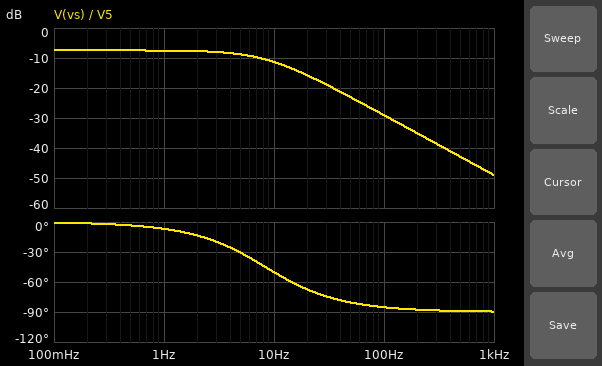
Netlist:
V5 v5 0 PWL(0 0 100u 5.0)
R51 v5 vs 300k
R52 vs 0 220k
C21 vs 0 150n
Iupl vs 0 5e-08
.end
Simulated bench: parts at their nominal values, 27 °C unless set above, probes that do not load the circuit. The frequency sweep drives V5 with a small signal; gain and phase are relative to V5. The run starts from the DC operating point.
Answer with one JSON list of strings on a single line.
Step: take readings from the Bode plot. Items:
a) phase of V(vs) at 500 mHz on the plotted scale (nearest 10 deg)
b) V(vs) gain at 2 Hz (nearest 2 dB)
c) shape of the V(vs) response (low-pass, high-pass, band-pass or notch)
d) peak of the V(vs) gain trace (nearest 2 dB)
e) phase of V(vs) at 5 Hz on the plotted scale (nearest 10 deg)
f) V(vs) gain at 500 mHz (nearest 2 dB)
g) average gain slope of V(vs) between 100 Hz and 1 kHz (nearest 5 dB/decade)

["0 deg", "-8 dB", "low-pass", "-8 dB", "-30 deg", "-8 dB", "-20 dB/decade"]
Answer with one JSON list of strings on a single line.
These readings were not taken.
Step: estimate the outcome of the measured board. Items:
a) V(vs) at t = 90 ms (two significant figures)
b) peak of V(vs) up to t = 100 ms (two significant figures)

["2.1 V", "2.1 V"]
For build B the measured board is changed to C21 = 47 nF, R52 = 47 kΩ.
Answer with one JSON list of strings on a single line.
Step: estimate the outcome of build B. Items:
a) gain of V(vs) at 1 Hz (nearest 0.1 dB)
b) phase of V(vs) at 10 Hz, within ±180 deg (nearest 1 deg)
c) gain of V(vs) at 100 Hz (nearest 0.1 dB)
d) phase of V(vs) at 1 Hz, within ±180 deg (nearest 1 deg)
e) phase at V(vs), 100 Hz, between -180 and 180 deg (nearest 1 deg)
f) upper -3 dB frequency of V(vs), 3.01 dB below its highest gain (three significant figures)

["-17.4 dB", "-7 deg", "-21.2 dB", "-1 deg", "-50 deg", "83.3 Hz"]
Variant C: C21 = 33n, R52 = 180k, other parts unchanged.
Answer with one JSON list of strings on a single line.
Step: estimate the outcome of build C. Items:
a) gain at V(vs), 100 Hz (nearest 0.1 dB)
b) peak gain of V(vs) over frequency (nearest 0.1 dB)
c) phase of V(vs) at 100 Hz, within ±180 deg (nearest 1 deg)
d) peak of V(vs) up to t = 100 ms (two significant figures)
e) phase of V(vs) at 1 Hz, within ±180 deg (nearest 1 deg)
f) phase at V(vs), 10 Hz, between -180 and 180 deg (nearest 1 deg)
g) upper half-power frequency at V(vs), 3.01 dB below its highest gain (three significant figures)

["-16.6 dB", "-8.5 dB", "-67 deg", "1.9 V", "-1 deg", "-13 deg", "42.9 Hz"]
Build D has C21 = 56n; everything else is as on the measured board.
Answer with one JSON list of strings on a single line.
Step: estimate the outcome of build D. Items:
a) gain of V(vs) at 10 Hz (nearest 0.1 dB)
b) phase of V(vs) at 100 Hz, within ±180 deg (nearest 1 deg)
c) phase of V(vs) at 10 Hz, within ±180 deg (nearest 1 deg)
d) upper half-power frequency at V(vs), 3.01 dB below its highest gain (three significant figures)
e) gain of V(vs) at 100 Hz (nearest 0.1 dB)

["-8.3 dB", "-77 deg", "-24 deg", "22.4 Hz", "-20.7 dB"]
